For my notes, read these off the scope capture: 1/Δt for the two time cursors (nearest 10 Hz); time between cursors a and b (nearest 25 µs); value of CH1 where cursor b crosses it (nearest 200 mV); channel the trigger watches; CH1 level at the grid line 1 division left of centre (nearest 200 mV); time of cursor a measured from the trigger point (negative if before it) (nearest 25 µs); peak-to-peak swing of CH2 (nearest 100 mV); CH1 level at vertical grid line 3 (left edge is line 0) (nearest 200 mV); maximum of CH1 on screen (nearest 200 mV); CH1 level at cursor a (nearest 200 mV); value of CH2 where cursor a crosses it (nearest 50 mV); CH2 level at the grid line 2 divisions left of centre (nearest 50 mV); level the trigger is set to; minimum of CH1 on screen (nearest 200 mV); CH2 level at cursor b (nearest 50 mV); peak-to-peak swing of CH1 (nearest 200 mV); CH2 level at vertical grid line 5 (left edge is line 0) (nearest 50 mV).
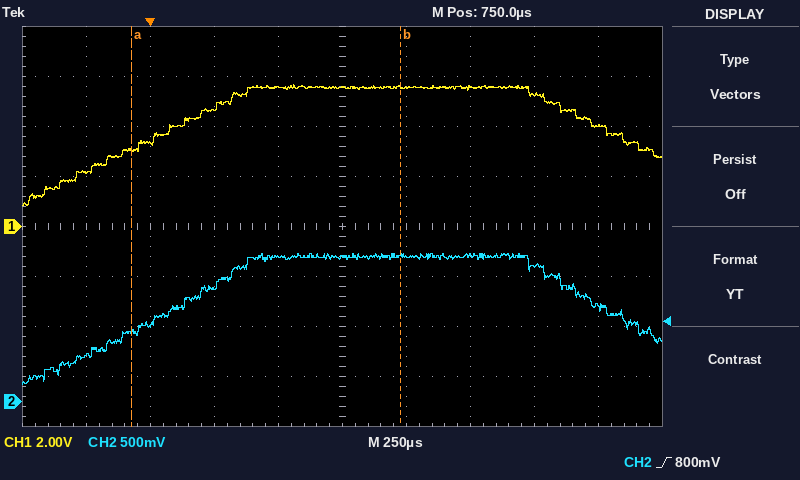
950 Hz
1.050 ms
5.6 V
CH2
5.6 V
-75 µs
1.30 V
4.8 V
5.6 V
3.0 V
700 mV
1.15 V
800 mV
800 mV
1.45 V
4.8 V
1.45 V
